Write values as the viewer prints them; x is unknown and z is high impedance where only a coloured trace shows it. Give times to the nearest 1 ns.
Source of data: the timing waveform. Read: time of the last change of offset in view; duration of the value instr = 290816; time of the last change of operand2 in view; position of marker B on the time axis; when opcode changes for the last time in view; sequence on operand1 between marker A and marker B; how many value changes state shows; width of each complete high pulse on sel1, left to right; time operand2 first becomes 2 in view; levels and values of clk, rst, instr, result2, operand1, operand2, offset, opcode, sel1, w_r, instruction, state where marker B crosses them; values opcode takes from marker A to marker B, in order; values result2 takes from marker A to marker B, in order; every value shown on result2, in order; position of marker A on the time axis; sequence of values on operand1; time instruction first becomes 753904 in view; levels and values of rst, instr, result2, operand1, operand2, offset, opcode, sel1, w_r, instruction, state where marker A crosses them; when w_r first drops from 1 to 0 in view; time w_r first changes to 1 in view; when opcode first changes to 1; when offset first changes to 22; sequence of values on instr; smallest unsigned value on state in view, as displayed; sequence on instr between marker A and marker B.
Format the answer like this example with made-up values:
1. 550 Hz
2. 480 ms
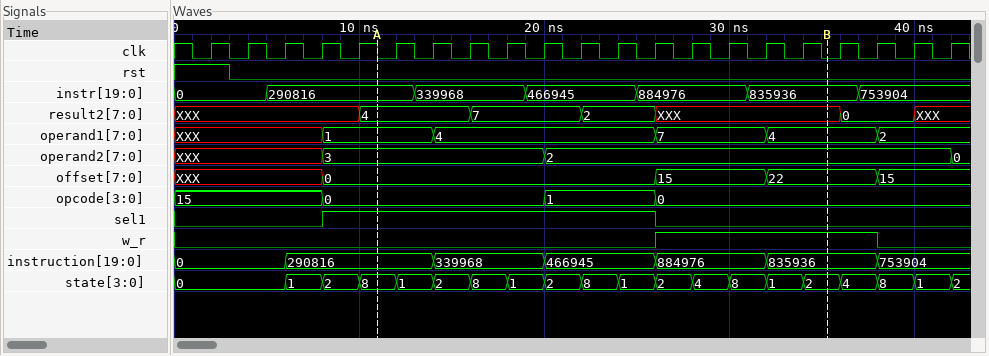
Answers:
1. 38 ns
2. 8 ns
3. 42 ns
4. 35 ns
5. 26 ns
6. 1, 4, 7, 4
7. 19
8. 18 ns
9. 20 ns
10. clk=0, rst=0, instr=835936, result2=XXX, operand1=4, operand2=2, offset=22, opcode=0, sel1=0, w_r=1, instruction=835936, state=2
11. 0, 1, 0
12. 4, 7, 2, XXX
13. XXX, 4, 7, 2, XXX, 0, XXX
14. 11 ns
15. XXX, 1, 4, 7, 4, 2
16. 38 ns
17. rst=0, instr=290816, result2=4, operand1=1, operand2=3, offset=0, opcode=0, sel1=1, w_r=0, instruction=290816, state=8
18. 38 ns
19. 26 ns
20. 20 ns
21. 32 ns
22. 0, 290816, 339968, 466945, 884976, 835936, 753904
23. 0
24. 290816, 339968, 466945, 884976, 835936
